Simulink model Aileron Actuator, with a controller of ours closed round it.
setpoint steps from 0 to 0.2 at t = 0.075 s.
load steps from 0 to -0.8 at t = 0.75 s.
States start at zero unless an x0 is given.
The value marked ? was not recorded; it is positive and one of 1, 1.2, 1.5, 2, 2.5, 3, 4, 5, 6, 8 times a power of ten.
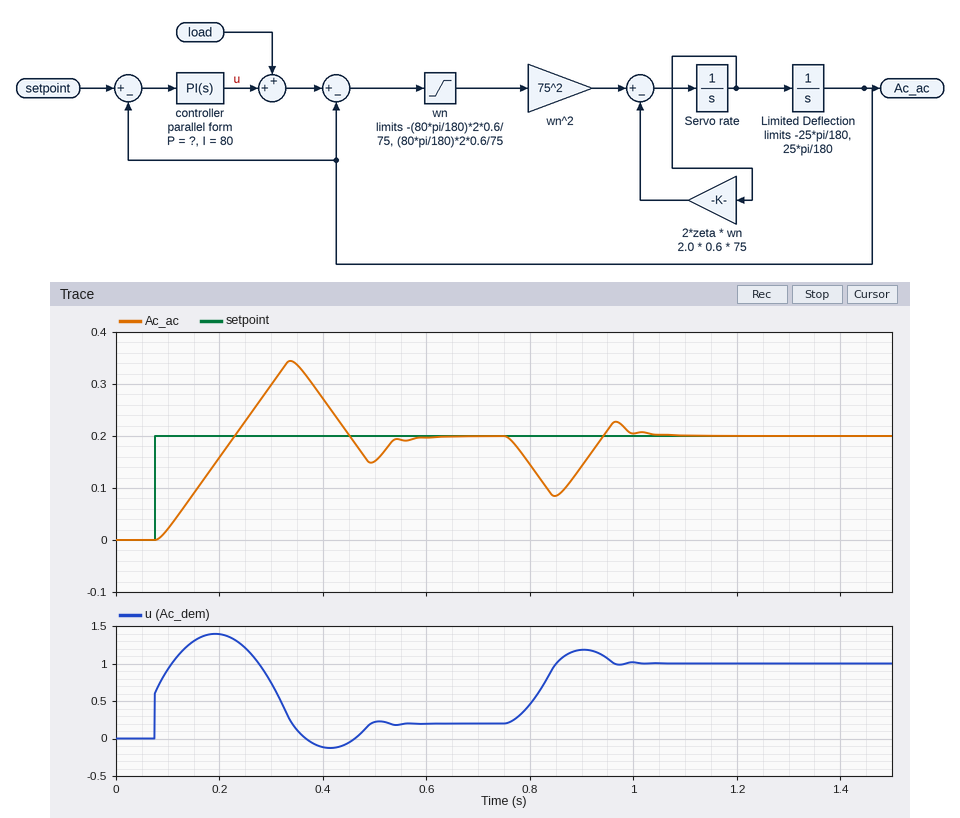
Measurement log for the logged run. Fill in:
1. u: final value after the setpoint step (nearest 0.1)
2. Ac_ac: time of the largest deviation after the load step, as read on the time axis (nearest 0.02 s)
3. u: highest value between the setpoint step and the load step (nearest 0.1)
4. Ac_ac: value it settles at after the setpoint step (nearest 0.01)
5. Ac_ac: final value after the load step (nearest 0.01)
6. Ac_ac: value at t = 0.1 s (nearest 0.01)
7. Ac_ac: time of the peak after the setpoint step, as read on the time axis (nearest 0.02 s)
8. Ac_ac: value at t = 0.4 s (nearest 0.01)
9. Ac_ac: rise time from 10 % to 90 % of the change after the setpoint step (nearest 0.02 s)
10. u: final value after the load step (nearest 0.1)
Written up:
0.2
0.84 s
1.4
0.20
0.20
0.02
0.34 s
0.27
0.12 s
1.0
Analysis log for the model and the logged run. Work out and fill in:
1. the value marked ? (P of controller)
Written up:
3
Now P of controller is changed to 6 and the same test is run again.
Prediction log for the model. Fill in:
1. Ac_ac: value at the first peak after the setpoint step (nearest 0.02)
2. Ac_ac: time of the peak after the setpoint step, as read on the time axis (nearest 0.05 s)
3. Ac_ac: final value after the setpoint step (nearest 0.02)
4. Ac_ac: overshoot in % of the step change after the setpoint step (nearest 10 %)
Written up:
0.32
0.30 s
0.20
60 %
